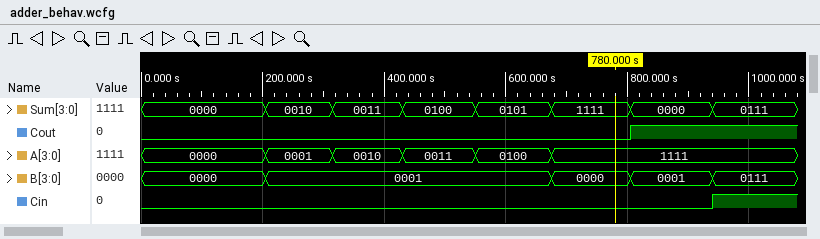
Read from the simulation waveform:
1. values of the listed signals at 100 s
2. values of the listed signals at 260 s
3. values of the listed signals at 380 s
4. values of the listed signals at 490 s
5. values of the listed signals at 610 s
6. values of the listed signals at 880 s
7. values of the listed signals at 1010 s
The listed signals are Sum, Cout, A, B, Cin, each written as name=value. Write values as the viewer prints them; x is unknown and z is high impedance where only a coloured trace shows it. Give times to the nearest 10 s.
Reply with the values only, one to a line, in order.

Sum=0000, Cout=0, A=0000, B=0000, Cin=0
Sum=0010, Cout=0, A=0001, B=0001, Cin=0
Sum=0011, Cout=0, A=0010, B=0001, Cin=0
Sum=0100, Cout=0, A=0011, B=0001, Cin=0
Sum=0101, Cout=0, A=0100, B=0001, Cin=0
Sum=0000, Cout=1, A=1111, B=0001, Cin=0
Sum=0111, Cout=1, A=1111, B=0111, Cin=1
